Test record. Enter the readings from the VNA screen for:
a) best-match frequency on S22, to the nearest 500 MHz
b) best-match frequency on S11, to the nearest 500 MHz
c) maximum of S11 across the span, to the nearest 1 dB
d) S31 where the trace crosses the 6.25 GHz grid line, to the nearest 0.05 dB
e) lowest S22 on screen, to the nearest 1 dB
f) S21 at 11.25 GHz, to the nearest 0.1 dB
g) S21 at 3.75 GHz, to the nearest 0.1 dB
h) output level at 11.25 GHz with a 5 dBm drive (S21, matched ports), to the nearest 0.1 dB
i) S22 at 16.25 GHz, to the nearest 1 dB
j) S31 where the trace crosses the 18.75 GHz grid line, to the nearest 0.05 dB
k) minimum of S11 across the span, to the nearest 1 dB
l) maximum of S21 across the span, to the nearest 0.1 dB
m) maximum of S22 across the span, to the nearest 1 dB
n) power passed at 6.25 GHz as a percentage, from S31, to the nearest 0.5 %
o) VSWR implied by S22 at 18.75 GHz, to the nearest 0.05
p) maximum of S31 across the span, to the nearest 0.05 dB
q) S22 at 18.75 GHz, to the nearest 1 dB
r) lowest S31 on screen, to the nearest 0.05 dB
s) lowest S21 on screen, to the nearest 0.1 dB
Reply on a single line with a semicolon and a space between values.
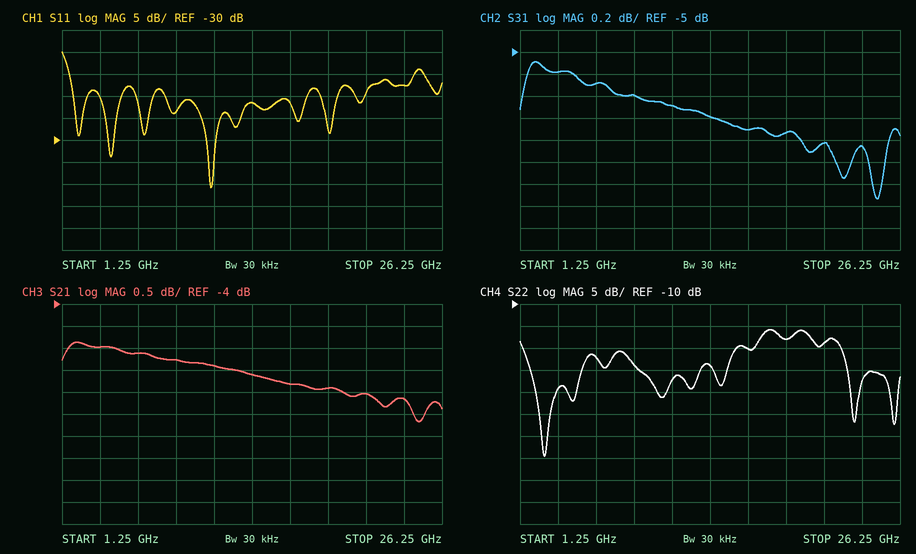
3.0 GHz; 11.0 GHz; -10 dB; -5.30 dB; -45 dB; -5.4 dB; -5.0 dB; -0.4 dBm; -20 dB; -5.75 dB; -41 dB; -4.9 dB; -16 dB; 29.5 %; 1.30; -5.10 dB; -18 dB; -6.35 dB; -6.7 dB
